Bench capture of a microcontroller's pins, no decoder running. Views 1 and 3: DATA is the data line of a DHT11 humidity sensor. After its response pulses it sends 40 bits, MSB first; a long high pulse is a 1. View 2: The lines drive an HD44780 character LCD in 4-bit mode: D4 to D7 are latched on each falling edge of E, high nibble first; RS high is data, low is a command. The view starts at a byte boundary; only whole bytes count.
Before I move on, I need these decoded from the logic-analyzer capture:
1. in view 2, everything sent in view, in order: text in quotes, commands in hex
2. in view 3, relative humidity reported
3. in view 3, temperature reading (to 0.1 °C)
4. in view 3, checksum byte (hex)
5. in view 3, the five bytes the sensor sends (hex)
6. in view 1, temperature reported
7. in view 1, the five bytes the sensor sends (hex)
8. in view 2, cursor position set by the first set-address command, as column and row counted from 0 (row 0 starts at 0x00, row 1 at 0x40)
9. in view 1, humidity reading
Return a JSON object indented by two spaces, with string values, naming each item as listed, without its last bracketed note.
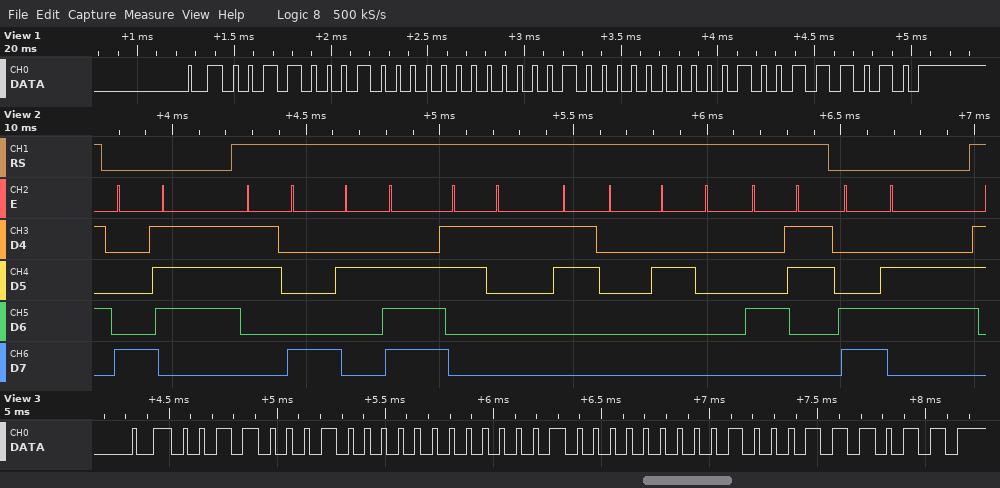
{
  "in view 2, everything sent in view, in order: text in quotes, commands in hex": "0x87 \"8.10 C\" 0xC6",
  "in view 3, relative humidity reported": "49 %",
  "in view 3, temperature reading": "8.2 °C",
  "in view 3, checksum byte": "0x3B",
  "in view 3, the five bytes the sensor sends": "31 00 08 02 3B",
  "in view 1, temperature reported": "8.1 °C",
  "in view 1, the five bytes the sensor sends": "31 00 08 01 3A",
  "in view 2, cursor position set by the first set-address command, as column and row counted from 0": "column 7, row 0",
  "in view 1, humidity reading": "49 %"
}
